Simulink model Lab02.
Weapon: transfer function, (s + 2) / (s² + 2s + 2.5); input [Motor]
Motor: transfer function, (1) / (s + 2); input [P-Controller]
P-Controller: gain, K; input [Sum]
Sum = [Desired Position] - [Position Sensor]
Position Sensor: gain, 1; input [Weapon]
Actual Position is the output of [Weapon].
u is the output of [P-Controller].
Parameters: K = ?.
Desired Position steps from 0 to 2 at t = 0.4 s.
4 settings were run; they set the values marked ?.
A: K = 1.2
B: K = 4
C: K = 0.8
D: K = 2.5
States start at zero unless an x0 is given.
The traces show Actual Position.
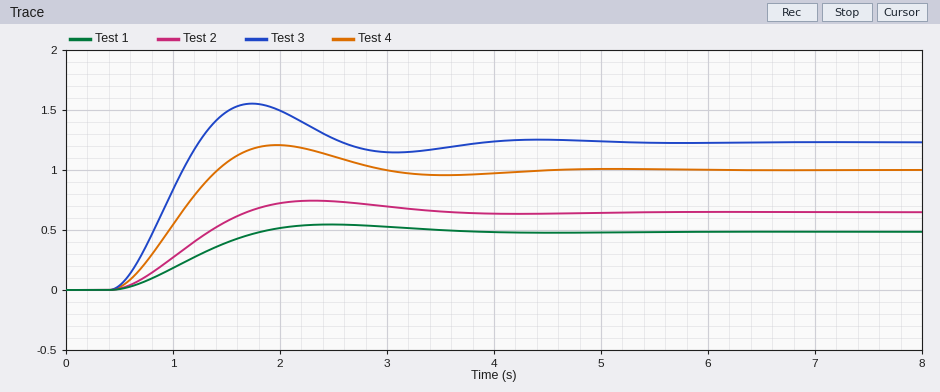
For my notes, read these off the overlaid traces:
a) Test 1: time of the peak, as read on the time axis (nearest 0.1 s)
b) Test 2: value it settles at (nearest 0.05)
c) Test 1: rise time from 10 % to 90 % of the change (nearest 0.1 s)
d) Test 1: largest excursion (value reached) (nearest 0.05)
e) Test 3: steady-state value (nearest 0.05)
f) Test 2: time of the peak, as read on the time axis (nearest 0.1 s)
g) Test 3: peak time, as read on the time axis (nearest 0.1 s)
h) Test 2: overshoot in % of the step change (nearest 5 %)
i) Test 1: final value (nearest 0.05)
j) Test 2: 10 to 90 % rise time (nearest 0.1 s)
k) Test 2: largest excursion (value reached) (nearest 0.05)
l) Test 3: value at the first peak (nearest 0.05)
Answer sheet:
2.5 s
0.65
1.0 s
0.55
1.25
2.3 s
1.7 s
15 %
0.50
0.9 s
0.75
1.55
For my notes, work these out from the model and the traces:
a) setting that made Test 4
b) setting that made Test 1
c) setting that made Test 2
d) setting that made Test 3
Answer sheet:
D
C
A
B
